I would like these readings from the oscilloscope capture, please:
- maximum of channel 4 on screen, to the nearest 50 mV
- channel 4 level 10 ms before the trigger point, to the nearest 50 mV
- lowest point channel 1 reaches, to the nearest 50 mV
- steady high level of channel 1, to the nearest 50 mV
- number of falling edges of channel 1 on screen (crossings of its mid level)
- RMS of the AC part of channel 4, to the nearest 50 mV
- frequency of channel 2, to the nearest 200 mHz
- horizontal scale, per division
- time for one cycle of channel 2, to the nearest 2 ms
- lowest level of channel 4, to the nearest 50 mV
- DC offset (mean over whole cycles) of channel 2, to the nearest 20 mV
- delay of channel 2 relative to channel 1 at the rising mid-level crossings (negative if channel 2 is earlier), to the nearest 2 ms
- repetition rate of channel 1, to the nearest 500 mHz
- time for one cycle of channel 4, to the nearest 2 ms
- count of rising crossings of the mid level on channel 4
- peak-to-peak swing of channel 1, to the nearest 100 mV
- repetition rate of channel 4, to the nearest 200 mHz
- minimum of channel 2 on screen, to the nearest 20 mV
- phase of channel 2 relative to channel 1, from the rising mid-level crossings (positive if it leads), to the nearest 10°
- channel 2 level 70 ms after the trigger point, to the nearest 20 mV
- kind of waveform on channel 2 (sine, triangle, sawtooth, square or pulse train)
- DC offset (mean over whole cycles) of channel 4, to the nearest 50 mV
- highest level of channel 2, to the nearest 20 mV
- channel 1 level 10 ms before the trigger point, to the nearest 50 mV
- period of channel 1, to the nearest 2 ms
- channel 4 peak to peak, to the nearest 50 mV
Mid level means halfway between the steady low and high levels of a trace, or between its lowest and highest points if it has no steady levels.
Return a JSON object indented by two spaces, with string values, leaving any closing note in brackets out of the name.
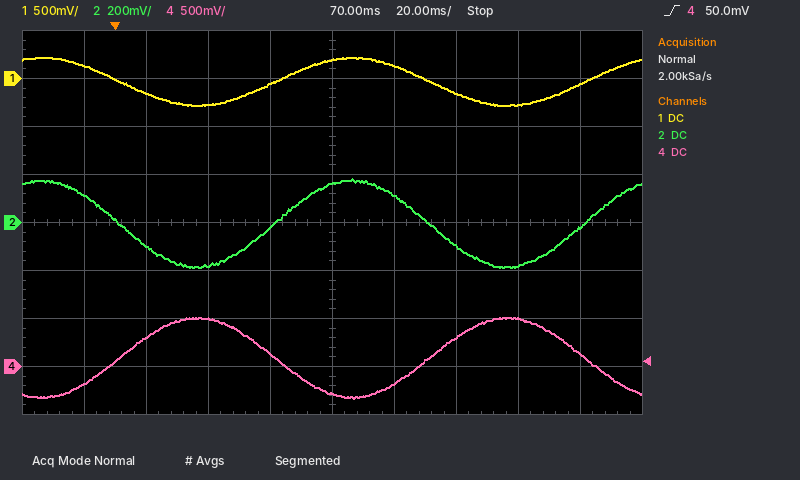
{
  "maximum of channel 4 on screen, to the nearest 50 mV": "500 mV",
  "channel 4 level 10 ms before the trigger point, to the nearest 50 mV": "-200 mV",
  "lowest point channel 1 reaches, to the nearest 50 mV": "-300 mV",
  "steady high level of channel 1, to the nearest 50 mV": "200 mV",
  "number of falling edges of channel 1 on screen": "2",
  "RMS of the AC part of channel 4, to the nearest 50 mV": "300 mV",
  "frequency of channel 2, to the nearest 200 mHz": "10.0 Hz",
  "horizontal scale, per division": "20 ms",
  "time for one cycle of channel 2, to the nearest 2 ms": "100 ms",
  "lowest level of channel 4, to the nearest 50 mV": "-350 mV",
  "DC offset (mean over whole cycles) of channel 2, to the nearest 20 mV": "0 mV",
  "delay of channel 2 relative to channel 1 at the rising mid-level crossings (negative if channel 2 is earlier), to the nearest 2 ms": "0 ms",
  "repetition rate of channel 1, to the nearest 500 mHz": "10.0 Hz",
  "time for one cycle of channel 4, to the nearest 2 ms": "100 ms",
  "count of rising crossings of the mid level on channel 4": "2",
  "peak-to-peak swing of channel 1, to the nearest 100 mV": "500 mV",
  "repetition rate of channel 4, to the nearest 200 mHz": "10.0 Hz",
  "minimum of channel 2 on screen, to the nearest 20 mV": "-180 mV",
  "phase of channel 2 relative to channel 1, from the rising mid-level crossings (positive if it leads), to the nearest 10°": "0°",
  "channel 2 level 70 ms after the trigger point, to the nearest 20 mV": "160 mV",
  "kind of waveform on channel 2": "sine",
  "DC offset (mean over whole cycles) of channel 4, to the nearest 50 mV": "100 mV",
  "highest level of channel 2, to the nearest 20 mV": "180 mV",
  "channel 1 level 10 ms before the trigger point, to the nearest 50 mV": "150 mV",
  "period of channel 1, to the nearest 2 ms": "100 ms",
  "channel 4 peak to peak, to the nearest 50 mV": "850 mV"
}
